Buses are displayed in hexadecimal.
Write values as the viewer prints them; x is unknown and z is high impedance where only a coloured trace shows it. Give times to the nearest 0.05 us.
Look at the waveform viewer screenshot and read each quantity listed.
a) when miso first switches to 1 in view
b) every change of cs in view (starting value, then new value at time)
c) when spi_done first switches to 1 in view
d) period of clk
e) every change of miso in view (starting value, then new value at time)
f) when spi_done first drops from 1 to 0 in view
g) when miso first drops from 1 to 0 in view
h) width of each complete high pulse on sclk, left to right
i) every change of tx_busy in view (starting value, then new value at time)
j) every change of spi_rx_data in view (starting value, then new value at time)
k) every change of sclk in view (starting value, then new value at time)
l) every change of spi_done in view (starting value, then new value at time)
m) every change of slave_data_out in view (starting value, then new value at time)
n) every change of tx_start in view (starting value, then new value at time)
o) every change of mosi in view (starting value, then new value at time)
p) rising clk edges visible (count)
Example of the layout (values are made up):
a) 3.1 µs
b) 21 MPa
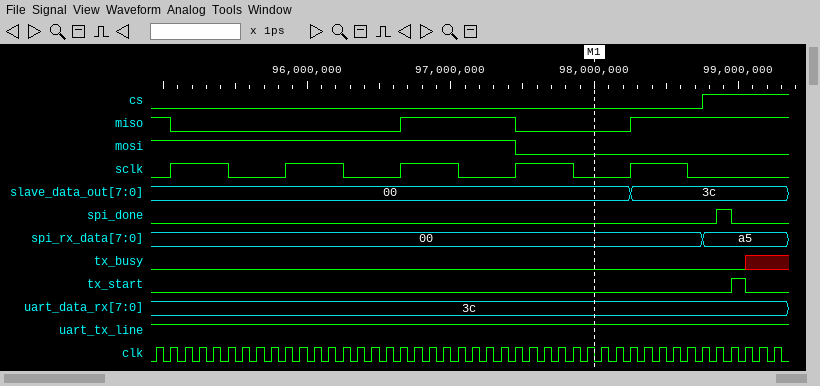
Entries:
a) 96.65 us
b) 0, 1 at 98.75 us
c) 98.85 us
d) 0.1 us
e) 1, 0 at 95.05 us, 1 at 96.65 us, 0 at 97.45 us, 1 at 98.25 us
f) 98.95 us
g) 95.05 us
h) 0.4 us, 0.4 us, 0.4 us, 0.4 us, 0.4 us
i) 0, x at 99.05 us
j) 00, a5 at 98.75 us
k) 0, 1 at 95.05 us, 0 at 95.45 us, 1 at 95.85 us, 0 at 96.25 us, 1 at 96.65 us, 0 at 97.05 us, 1 at 97.45 us, 0 at 97.85 us, 1 at 98.25 us, 0 at 98.65 us
l) 0, 1 at 98.85 us, 0 at 98.95 us
m) 00, 3c at 98.25 us
n) 0, 1 at 98.95 us, 0 at 99.05 us
o) 1, 0 at 97.45 us
p) 44
